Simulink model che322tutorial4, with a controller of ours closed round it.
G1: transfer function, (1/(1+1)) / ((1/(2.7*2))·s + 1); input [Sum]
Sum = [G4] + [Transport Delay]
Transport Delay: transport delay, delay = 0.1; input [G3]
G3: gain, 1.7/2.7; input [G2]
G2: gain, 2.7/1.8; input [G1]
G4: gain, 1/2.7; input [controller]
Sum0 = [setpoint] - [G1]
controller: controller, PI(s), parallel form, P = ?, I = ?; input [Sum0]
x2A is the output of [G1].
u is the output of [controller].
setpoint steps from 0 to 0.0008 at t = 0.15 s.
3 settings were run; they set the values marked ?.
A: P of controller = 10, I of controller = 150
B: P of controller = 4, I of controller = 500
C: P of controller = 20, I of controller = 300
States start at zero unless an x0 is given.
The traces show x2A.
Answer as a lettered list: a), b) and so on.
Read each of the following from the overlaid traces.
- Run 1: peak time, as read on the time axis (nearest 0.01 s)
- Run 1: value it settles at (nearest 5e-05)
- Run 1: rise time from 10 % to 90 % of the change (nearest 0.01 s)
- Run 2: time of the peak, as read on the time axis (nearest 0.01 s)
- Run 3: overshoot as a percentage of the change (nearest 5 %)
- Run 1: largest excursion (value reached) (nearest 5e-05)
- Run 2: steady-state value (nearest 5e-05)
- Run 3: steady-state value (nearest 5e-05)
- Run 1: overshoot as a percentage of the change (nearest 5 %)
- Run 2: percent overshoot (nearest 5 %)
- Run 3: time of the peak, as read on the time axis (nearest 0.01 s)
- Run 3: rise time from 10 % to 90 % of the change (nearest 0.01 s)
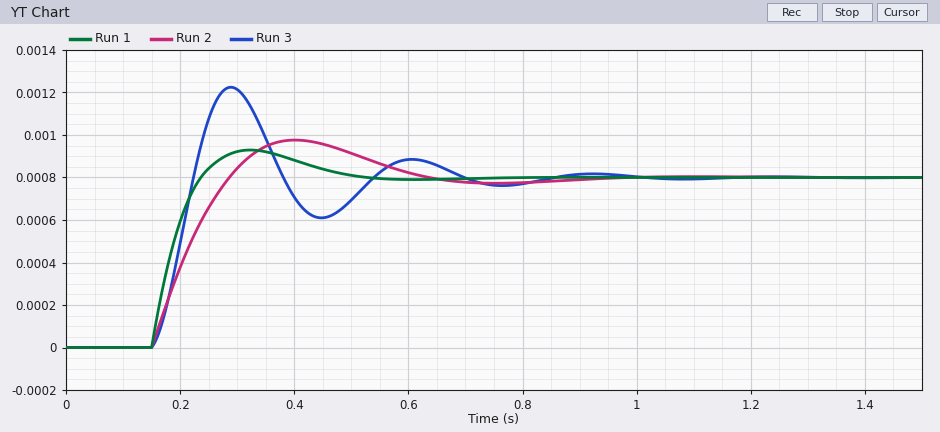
a) 0.32 s
b) 0.00080
c) 0.06 s
d) 0.40 s
e) 55 %
f) 0.00095
g) 0.00080
h) 0.00080
i) 15 %
j) 20 %
k) 0.29 s
l) 0.05 s
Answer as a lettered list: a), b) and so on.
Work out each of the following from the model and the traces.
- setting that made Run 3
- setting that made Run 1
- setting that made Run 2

a) B
b) C
c) A
